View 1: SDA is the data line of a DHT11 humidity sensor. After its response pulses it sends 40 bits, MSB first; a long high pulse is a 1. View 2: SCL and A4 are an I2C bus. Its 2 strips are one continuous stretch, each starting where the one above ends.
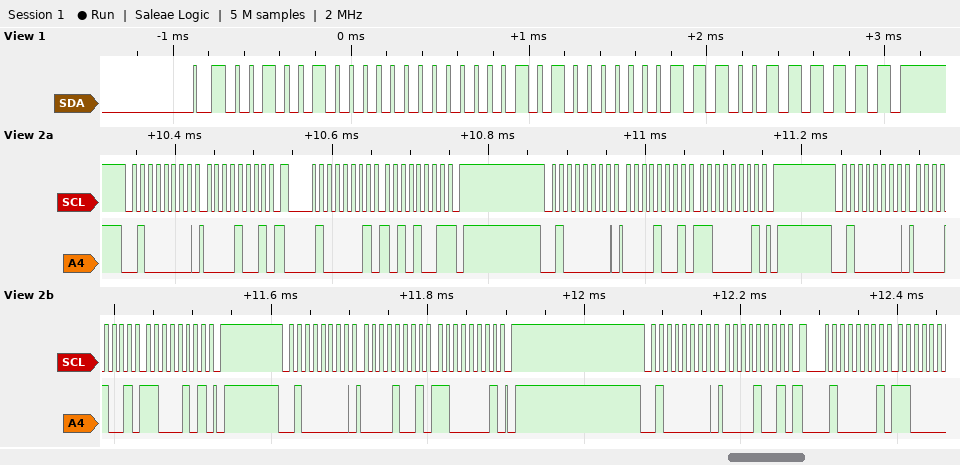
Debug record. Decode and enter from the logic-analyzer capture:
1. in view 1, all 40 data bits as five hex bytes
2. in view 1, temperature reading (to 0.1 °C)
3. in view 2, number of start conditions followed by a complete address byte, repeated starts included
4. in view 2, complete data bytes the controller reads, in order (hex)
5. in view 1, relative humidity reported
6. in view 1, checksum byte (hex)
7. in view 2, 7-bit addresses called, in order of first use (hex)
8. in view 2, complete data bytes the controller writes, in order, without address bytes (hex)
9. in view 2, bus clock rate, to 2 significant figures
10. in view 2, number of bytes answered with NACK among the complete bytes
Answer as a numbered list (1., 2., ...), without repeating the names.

1. 24 00 14 07 3F
2. 20.7 °C
3. 7
4. A9
5. 36 %
6. 0x3F
7. 0x20
8. 09 09 C1 09 C5 09 C1 09
9. 100 kHz
10. 1
